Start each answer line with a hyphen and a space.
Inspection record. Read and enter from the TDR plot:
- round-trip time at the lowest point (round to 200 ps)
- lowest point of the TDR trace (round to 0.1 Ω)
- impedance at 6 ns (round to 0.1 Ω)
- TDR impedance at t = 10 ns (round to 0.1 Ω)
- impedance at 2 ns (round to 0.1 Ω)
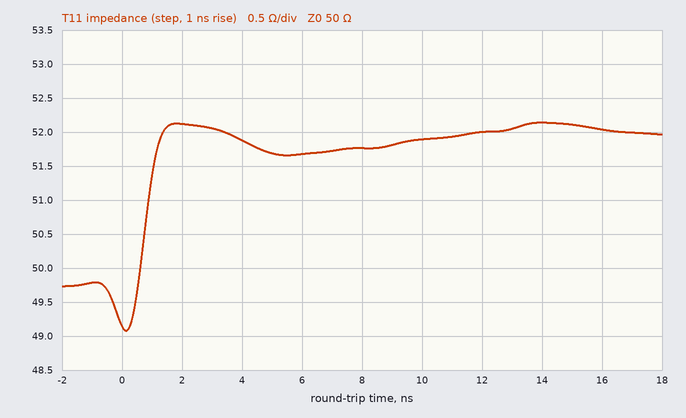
- 200 ps
- 49.1 Ω
- 51.7 Ω
- 51.9 Ω
- 52.1 Ω
